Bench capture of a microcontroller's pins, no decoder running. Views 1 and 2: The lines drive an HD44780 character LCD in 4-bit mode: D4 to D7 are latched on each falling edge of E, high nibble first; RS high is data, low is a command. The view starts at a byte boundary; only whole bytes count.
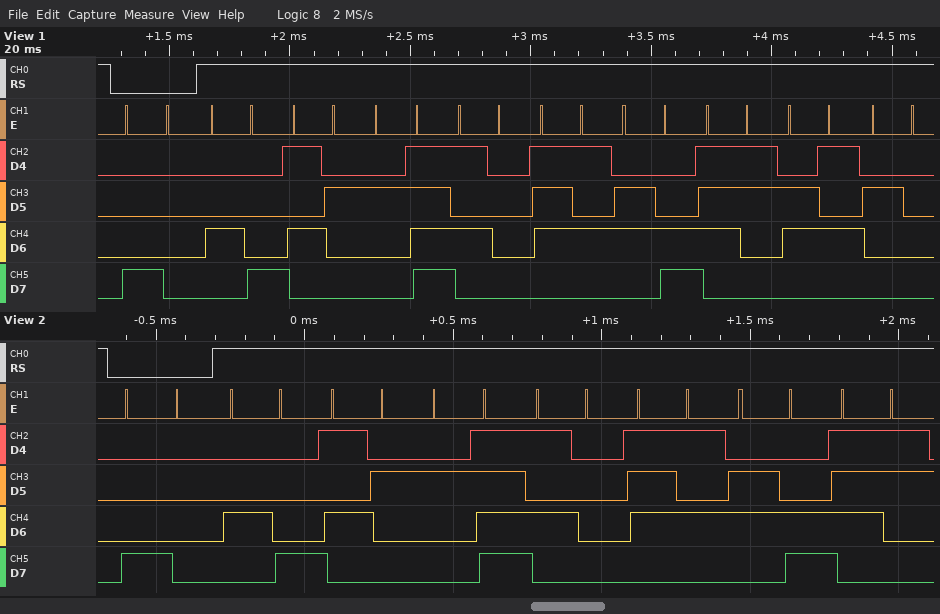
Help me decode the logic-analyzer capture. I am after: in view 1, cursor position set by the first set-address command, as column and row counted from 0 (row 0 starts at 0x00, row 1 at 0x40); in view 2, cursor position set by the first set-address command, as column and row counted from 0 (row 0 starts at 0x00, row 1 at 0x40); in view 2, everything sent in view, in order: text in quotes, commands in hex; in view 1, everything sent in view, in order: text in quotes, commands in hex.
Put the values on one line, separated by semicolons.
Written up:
column 0, row 0; column 0, row 0; 0x80 "HR/Puls"; 0x80 "HR/Pulse "
